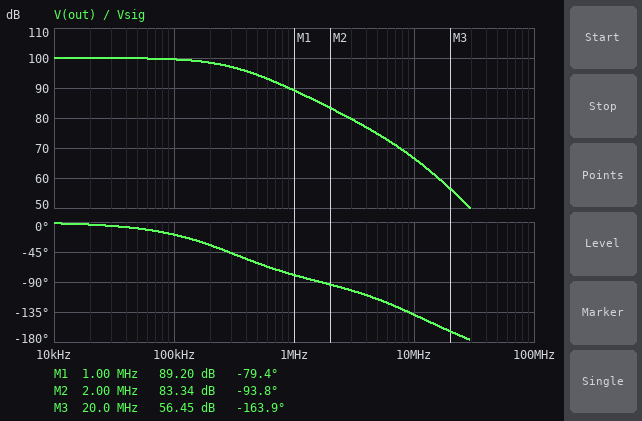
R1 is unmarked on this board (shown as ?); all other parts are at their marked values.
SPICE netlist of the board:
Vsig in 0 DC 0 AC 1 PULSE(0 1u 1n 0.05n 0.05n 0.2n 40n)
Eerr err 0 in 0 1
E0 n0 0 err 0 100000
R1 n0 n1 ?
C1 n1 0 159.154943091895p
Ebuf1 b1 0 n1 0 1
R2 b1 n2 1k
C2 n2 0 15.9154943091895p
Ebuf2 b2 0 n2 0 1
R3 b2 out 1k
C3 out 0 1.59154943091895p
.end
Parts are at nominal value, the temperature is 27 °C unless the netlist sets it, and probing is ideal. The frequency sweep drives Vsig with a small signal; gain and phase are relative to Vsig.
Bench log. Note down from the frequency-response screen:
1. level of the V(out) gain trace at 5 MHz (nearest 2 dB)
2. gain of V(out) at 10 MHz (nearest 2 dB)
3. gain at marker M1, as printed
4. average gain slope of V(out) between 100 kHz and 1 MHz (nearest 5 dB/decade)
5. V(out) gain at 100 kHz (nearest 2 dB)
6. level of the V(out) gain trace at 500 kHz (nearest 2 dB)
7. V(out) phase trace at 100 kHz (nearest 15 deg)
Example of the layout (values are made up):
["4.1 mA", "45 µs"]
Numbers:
["74 dB", "66 dB", "89.20 dB", "-10 dB/decade", "100 dB", "94 dB", "-15 deg"]
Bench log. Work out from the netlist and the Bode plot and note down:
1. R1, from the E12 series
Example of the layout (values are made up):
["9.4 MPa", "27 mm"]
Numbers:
["3.3 kΩ"]
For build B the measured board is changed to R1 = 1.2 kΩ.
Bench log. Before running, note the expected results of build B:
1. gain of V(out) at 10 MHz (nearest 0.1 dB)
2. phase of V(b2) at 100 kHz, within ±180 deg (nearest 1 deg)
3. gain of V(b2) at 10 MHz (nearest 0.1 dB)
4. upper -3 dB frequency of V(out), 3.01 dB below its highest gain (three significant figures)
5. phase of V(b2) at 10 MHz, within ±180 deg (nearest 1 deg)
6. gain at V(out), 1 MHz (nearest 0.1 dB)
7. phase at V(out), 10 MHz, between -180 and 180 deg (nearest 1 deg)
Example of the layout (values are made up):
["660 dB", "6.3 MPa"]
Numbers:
["75.3 dB", "-7 deg", "75.4 dB", "828 kHz", "-130 deg", "96.1 dB", "-136 deg"]
